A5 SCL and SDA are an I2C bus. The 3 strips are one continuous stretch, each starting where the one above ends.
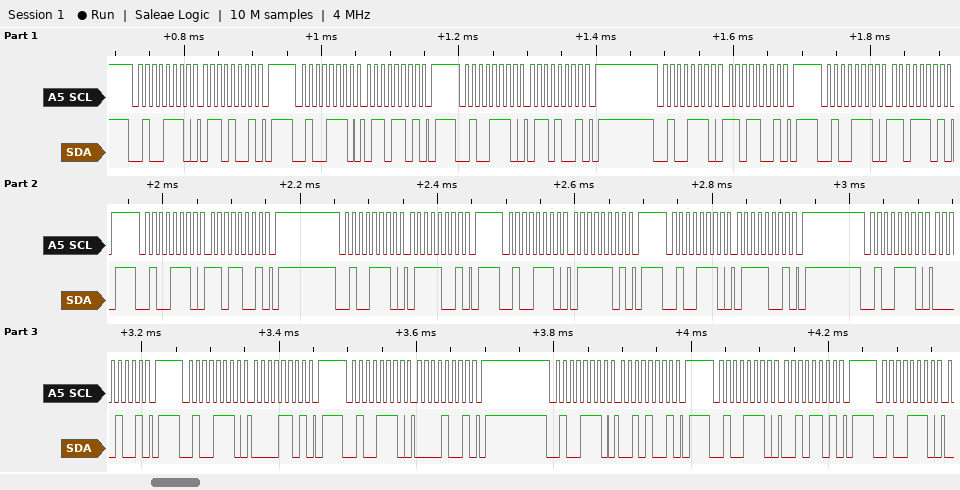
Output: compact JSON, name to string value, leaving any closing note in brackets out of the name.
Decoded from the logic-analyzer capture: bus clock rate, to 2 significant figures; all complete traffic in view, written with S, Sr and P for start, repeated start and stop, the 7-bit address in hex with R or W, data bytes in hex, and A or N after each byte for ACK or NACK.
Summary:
{"bus clock rate, to 2 significant figures": "100 kHz", "all complete traffic in view, written with S, Sr and P for start, repeated start and stop, the 7-bit address in hex with R or W, data bytes in hex, and A or N after each byte for ACK or NACK": "S 27W A 69 A P S 27W A 6D A P S 27W A 69 A P S 27W A D9 A P S 27W A DD A P S 27W A D9 A P S 27W A 79 A P S 27W A 7D A P S 27W A 79 A P S 27W A 09 A P S 27W A 0D A P S 27W A 09 A P S 27W A 29 A P S 27W A 2D A P S 27W A"}
